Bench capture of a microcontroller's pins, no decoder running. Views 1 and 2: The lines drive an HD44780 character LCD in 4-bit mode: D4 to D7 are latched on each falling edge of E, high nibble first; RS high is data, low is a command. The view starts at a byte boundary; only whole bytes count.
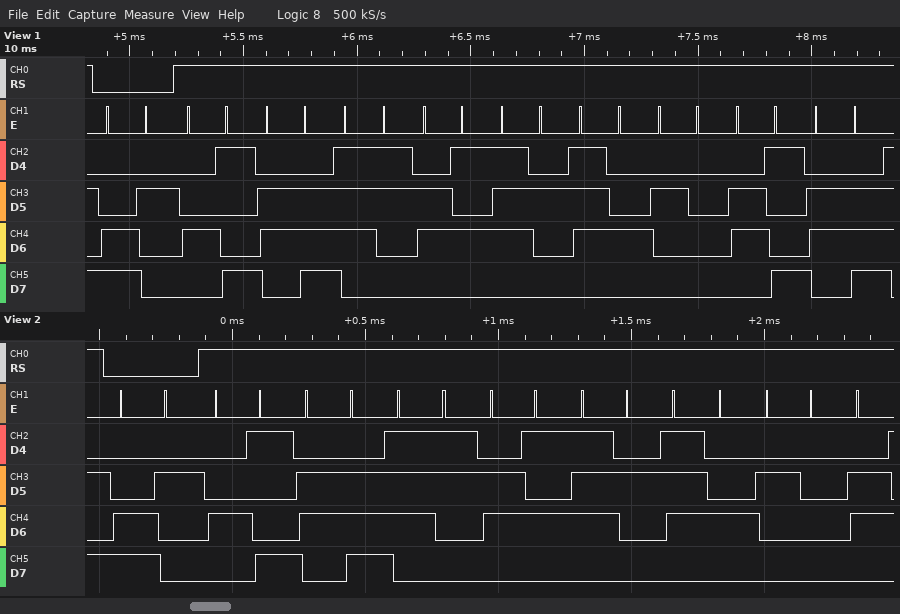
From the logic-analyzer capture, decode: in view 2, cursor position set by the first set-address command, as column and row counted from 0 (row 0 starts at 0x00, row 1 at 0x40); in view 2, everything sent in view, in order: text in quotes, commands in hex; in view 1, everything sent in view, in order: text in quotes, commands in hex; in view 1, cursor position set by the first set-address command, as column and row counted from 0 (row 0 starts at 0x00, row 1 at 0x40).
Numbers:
column 2, row 1
0xC2 "Insert "
0xC2 "Insert in"
column 2, row 1
